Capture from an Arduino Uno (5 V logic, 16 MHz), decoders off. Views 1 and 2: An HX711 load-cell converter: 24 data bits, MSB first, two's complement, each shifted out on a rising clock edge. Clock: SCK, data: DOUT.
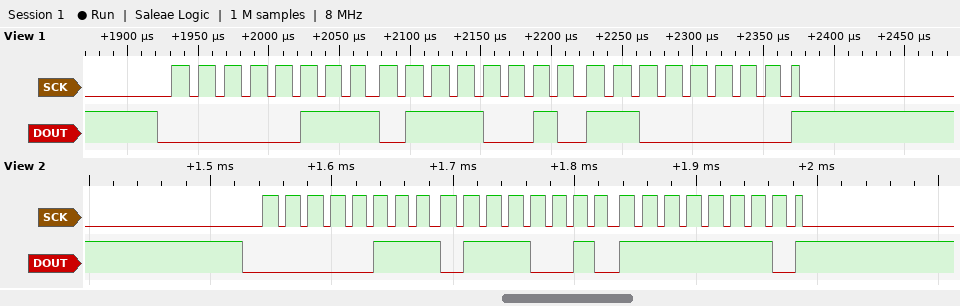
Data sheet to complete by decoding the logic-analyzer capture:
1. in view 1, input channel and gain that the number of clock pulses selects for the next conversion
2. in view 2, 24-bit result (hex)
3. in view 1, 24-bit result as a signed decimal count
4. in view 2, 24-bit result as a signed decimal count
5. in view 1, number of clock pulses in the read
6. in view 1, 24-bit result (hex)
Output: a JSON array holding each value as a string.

["channel A, gain 128", "0x0772FE", "488128", "488190", "25", "0x0772C0"]
